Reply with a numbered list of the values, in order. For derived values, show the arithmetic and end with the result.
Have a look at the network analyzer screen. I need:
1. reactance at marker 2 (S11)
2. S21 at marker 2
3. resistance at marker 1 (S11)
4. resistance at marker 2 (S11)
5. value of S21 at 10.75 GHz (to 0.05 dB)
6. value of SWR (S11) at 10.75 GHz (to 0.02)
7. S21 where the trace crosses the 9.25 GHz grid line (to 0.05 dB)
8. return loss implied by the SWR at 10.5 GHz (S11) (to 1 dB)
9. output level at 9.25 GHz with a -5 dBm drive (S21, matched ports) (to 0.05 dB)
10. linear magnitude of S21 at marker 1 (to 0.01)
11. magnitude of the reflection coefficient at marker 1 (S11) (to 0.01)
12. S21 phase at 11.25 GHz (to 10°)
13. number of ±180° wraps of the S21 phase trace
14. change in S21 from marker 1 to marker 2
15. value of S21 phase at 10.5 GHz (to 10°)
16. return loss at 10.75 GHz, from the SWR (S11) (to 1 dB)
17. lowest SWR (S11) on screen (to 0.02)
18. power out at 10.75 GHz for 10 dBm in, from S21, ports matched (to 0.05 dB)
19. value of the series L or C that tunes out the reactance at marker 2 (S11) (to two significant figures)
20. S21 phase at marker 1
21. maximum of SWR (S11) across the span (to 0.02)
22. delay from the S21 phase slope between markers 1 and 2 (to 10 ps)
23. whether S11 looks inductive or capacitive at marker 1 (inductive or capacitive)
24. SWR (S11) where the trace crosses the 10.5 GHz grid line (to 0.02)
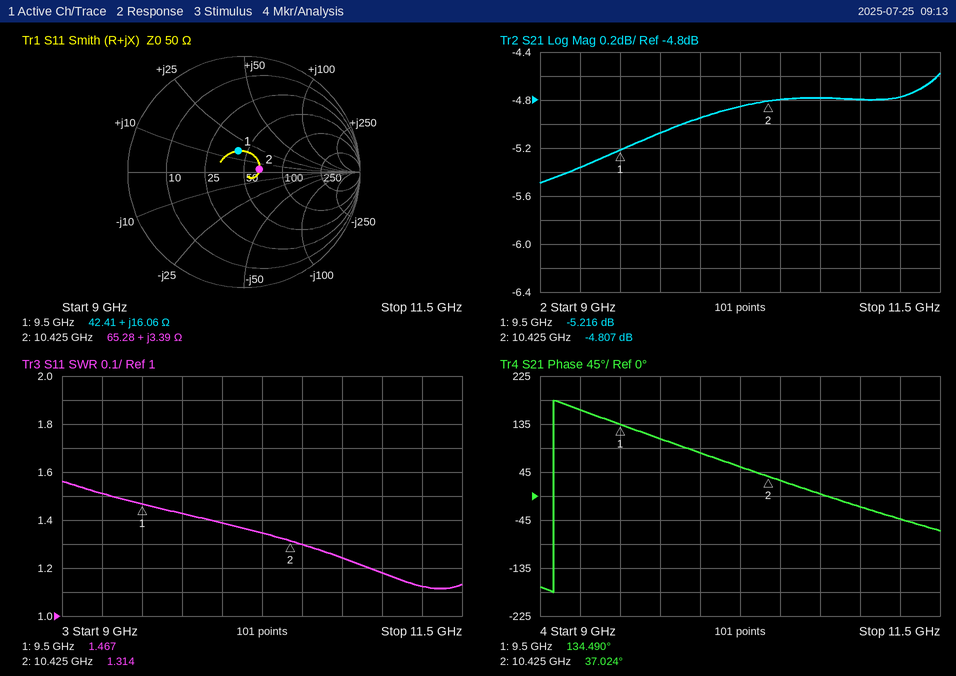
1. +3.39 Ω
2. -4.807 dB
3. 42.41 Ω
4. 65.28 Ω
5. -4.80 dB
6. 1.24
7. -5.35 dB
8. −20 log10((1.3 − 1)/(1.3 + 1)) ≈ 18 dB
9. -5 dBm + (-5.35 dB) = -10.35 dBm
10. 10^(-5.216/20) ≈ 0.55
11. 0.19
12. -40°
13. 1
14. -4.807 − (-5.216) = 0.409 dB
15. 30°
16. −20 log10((1.24 − 1)/(1.24 + 1)) ≈ 19 dB
17. 1.12
18. 10 dBm + (-4.80 dB) = 5.20 dBm
19. C = 1/(2π × 10.425 GHz × 3.39 Ω) ≈ 4.5 pF
20. 134.490°
21. 1.56
22. −(37.024° − (134.49°))/(360° × 925 MHz) ≈ 293 ps, so 290 ps to the nearest 10 ps
23. inductive
24. 1.30
